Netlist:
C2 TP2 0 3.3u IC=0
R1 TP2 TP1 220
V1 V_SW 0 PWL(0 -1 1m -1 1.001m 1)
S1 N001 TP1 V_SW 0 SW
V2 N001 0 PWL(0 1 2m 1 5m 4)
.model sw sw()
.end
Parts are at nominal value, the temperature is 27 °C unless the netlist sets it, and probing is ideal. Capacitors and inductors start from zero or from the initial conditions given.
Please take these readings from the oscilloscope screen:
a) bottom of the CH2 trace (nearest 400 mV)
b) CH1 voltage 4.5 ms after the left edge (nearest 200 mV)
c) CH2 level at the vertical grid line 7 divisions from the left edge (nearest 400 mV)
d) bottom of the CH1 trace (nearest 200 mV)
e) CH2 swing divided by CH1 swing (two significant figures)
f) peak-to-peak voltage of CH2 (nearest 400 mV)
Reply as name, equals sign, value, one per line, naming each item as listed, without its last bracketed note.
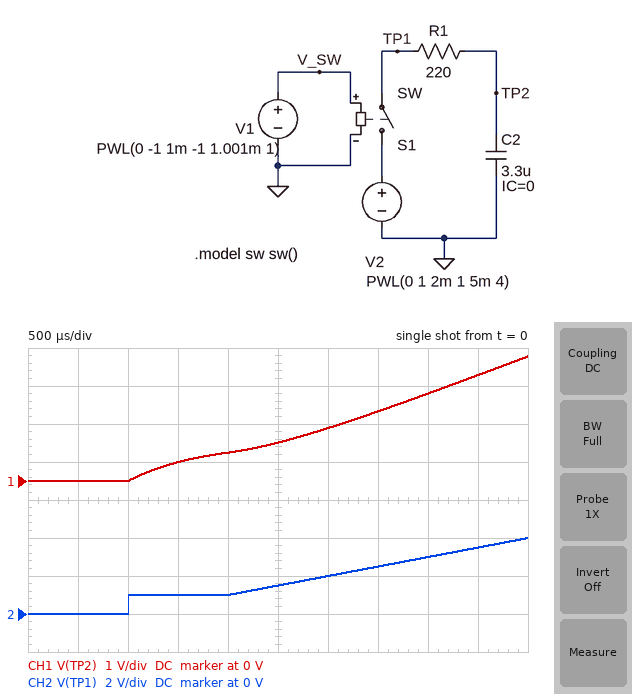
bottom of the CH2 trace = 0 V
CH1 voltage 4.5 ms after the left edge = 2.8 V
CH2 level at the vertical grid line 7 divisions from the left edge = 2.4 V
bottom of the CH1 trace = 0 V
CH2 swing divided by CH1 swing = 1.2
peak-to-peak voltage of CH2 = 4.0 V
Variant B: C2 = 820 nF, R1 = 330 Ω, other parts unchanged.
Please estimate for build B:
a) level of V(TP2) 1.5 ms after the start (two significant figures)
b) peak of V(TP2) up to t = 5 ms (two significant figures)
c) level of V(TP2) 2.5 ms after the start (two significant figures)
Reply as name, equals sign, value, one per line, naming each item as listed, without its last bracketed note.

level of V(TP2) 1.5 ms after the start = 840 mV
peak of V(TP2) up to t = 5 ms = 3.7 V
level of V(TP2) 2.5 ms after the start = 1.3 V
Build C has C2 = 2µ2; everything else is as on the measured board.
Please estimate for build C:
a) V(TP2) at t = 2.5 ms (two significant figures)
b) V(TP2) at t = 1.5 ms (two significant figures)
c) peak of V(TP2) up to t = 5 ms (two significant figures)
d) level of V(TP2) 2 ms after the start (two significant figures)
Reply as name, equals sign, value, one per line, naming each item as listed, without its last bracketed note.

V(TP2) at t = 2.5 ms = 1.1 V
V(TP2) at t = 1.5 ms = 640 mV
peak of V(TP2) up to t = 5 ms = 3.5 V
level of V(TP2) 2 ms after the start = 870 mV
